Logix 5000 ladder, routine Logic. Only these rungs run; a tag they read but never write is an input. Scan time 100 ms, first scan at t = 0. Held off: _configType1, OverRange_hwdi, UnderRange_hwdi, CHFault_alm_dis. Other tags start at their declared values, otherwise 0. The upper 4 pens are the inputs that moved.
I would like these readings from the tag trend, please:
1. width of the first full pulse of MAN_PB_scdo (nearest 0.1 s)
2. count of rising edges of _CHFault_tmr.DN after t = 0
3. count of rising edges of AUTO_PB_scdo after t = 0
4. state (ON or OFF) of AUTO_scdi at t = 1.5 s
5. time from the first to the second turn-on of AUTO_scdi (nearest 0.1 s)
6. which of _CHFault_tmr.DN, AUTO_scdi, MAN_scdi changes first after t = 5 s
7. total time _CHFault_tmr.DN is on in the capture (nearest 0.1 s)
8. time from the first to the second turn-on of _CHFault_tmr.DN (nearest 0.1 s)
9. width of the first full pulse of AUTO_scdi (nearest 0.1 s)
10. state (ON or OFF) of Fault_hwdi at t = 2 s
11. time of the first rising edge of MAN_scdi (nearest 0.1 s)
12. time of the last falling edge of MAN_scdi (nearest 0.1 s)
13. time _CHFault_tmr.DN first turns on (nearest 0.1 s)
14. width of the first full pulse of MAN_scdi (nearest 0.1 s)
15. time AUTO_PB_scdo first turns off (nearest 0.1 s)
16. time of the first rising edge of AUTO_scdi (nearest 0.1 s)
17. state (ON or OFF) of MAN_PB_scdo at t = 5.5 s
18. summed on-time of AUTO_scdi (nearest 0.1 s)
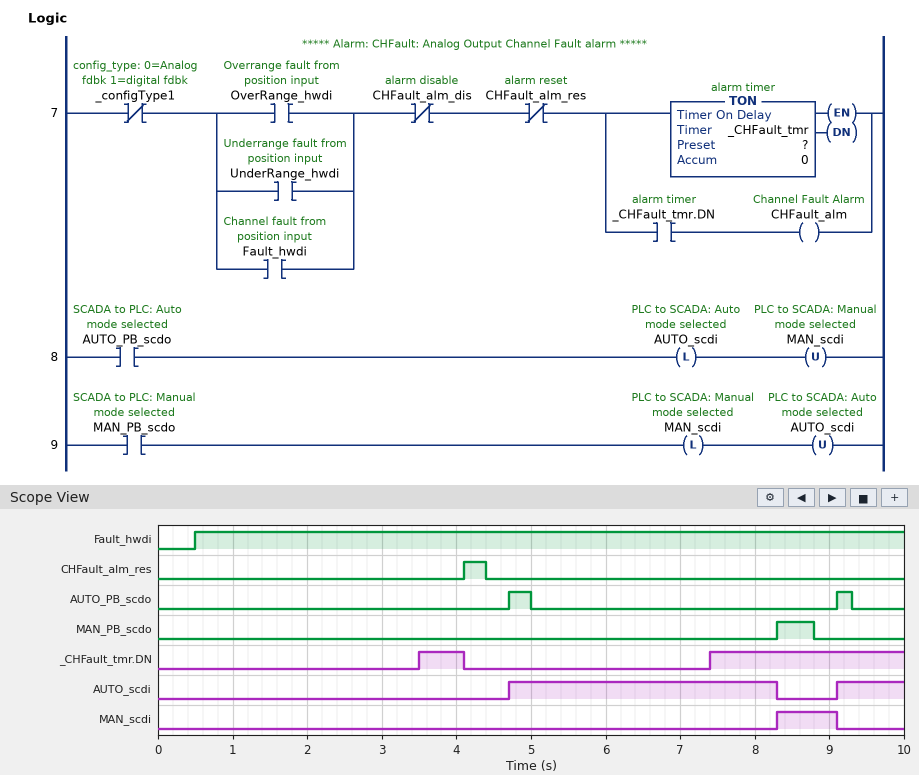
0.5 s
2
2
OFF
4.4 s
_CHFault_tmr.DN
3.2 s
3.9 s
3.6 s
ON
8.3 s
9.1 s
3.5 s
0.8 s
5.0 s
4.7 s
OFF
4.5 s
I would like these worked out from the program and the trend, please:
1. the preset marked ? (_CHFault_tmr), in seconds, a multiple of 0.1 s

3.0 s
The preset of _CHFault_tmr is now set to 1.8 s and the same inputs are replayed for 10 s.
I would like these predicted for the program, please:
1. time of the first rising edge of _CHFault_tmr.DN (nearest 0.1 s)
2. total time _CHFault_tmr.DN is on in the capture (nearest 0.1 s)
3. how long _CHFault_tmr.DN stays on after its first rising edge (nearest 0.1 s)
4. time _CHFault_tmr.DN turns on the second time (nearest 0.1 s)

2.3 s
5.6 s
1.8 s
6.2 s
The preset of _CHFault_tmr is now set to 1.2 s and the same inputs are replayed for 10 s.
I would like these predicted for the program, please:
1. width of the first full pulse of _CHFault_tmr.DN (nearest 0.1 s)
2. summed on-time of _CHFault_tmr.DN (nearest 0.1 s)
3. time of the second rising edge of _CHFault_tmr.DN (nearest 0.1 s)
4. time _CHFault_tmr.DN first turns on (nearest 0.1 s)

2.4 s
6.8 s
5.6 s
1.7 s
